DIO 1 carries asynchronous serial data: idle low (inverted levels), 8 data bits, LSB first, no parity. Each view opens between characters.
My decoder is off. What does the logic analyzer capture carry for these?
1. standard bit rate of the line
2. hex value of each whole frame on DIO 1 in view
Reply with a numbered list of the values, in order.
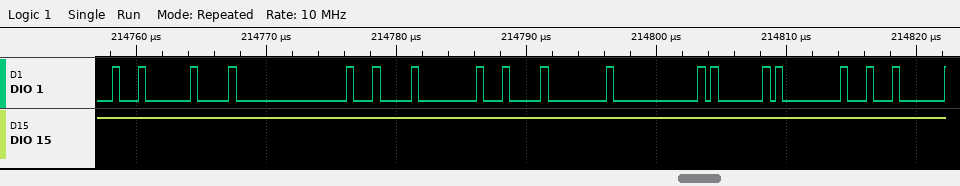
1. 2000000 baud
2. F7, DF, F7, FF, F7, FF, FF, FD, FD, 77
